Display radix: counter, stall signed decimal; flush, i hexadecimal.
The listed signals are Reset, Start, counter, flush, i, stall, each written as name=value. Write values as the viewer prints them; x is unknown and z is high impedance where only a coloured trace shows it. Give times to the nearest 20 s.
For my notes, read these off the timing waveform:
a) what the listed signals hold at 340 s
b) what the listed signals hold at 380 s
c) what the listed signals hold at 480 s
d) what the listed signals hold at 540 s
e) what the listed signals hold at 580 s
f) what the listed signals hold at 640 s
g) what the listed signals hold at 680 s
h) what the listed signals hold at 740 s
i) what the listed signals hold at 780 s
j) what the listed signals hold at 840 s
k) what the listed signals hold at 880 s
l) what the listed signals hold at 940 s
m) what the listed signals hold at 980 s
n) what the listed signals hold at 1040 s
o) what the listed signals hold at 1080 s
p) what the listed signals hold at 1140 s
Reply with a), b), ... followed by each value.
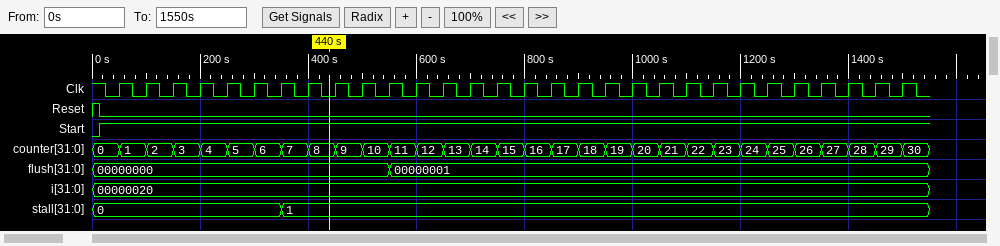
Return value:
a) Reset=0, Start=1, counter=6, flush=00000000, i=00000020, stall=0
b) Reset=0, Start=1, counter=7, flush=00000000, i=00000020, stall=1
c) Reset=0, Start=1, counter=9, flush=00000000, i=00000020, stall=1
d) Reset=0, Start=1, counter=10, flush=00000000, i=00000020, stall=1
e) Reset=0, Start=1, counter=11, flush=00000001, i=00000020, stall=1
f) Reset=0, Start=1, counter=12, flush=00000001, i=00000020, stall=1
g) Reset=0, Start=1, counter=13, flush=00000001, i=00000020, stall=1
h) Reset=0, Start=1, counter=14, flush=00000001, i=00000020, stall=1
i) Reset=0, Start=1, counter=15, flush=00000001, i=00000020, stall=1
j) Reset=0, Start=1, counter=16, flush=00000001, i=00000020, stall=1
k) Reset=0, Start=1, counter=17, flush=00000001, i=00000020, stall=1
l) Reset=0, Start=1, counter=18, flush=00000001, i=00000020, stall=1
m) Reset=0, Start=1, counter=19, flush=00000001, i=00000020, stall=1
n) Reset=0, Start=1, counter=20, flush=00000001, i=00000020, stall=1
o) Reset=0, Start=1, counter=21, flush=00000001, i=00000020, stall=1
p) Reset=0, Start=1, counter=22, flush=00000001, i=00000020, stall=1
